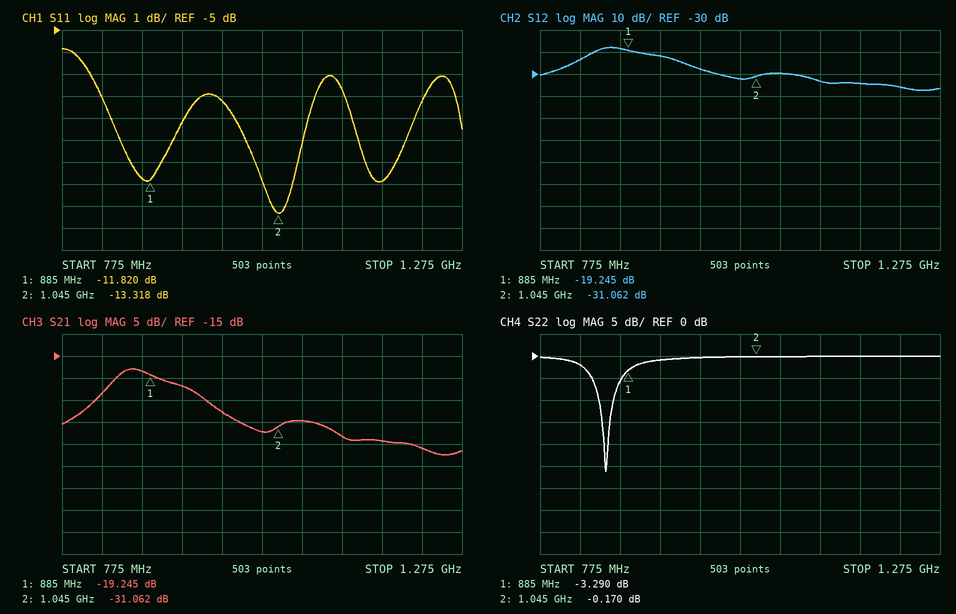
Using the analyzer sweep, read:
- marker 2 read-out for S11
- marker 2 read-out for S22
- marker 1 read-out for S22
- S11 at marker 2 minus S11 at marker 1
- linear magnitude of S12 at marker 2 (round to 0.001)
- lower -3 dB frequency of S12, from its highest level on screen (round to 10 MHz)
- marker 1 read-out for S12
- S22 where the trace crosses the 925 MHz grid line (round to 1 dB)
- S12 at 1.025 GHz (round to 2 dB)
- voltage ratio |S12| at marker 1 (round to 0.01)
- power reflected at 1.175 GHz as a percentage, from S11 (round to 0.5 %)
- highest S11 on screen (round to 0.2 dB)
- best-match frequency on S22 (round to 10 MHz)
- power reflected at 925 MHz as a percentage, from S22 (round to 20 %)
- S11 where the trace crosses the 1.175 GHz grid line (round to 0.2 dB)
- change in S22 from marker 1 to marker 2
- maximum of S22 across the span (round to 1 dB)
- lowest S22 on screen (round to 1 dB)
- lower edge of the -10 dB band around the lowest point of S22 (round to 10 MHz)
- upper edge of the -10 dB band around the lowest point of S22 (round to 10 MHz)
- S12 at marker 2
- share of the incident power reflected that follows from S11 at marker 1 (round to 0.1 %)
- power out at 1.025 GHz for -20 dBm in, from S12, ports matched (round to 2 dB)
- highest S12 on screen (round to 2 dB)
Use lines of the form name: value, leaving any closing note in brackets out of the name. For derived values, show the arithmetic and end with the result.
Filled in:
marker 2 read-out for S11: -13.318 dB
marker 2 read-out for S22: -0.170 dB
marker 1 read-out for S22: -3.290 dB
S11 at marker 2 minus S11 at marker 1: -13.318 − (-11.82) = -1.498 dB
linear magnitude of S12 at marker 2: 10^(-31.062/20) ≈ 0.028
lower -3 dB frequency of S12, from its highest level on screen: 840 MHz
marker 1 read-out for S12: -19.245 dB
S22 where the trace crosses the 925 MHz grid line: -1 dB
S12 at 1.025 GHz: -32 dB
voltage ratio |S12| at marker 1: 10^(-19.245/20) ≈ 0.11
power reflected at 1.175 GHz as a percentage, from S11: 10^(-11.8/10) ≈ 6.61 %, so 6.5 % to the nearest 0.5 %
highest S11 on screen: -5.8 dB
best-match frequency on S22: 860 MHz
power reflected at 925 MHz as a percentage, from S22: 10^(-1/10) ≈ 79.4 %, so 80 % to the nearest 20 %
S11 where the trace crosses the 1.175 GHz grid line: -11.8 dB
change in S22 from marker 1 to marker 2: -0.17 − (-3.29) = 3.120 dB
maximum of S22 across the span: 0 dB
lowest S22 on screen: -26 dB
lower edge of the -10 dB band around the lowest point of S22: 850 MHz
upper edge of the -10 dB band around the lowest point of S22: 870 MHz
S12 at marker 2: -31.062 dB
share of the incident power reflected that follows from S11 at marker 1: 10^(-11.82/10) ≈ 6.6 %
power out at 1.025 GHz for -20 dBm in, from S12, ports matched: -20 dBm + (-32 dB) = -52 dBm
highest S12 on screen: -18 dB
